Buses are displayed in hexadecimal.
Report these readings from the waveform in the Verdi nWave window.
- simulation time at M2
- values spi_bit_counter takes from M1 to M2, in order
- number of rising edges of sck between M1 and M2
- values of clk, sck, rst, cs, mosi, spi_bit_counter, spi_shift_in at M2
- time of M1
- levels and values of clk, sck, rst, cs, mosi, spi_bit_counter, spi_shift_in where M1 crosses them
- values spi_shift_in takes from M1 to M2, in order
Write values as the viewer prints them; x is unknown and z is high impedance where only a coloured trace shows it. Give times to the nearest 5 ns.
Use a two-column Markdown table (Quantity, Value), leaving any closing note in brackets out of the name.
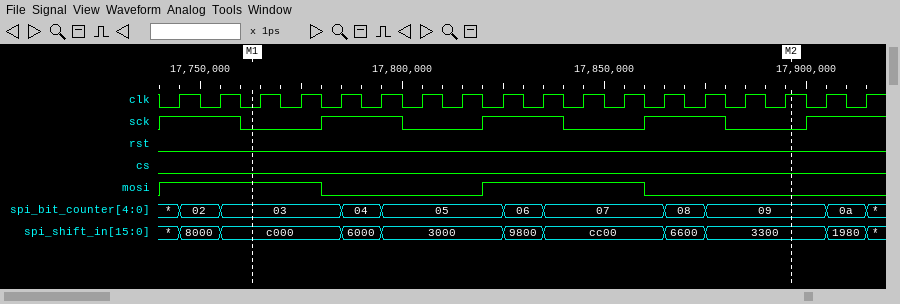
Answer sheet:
| Quantity | Value |
|---|---|
| simulation time at M2 | 17895 ns |
| values spi_bit_counter takes from M1 to M2, in order | 03, 04, 05, 06, 07, 08, 09 |
| number of rising edges of sck between M1 and M2 | 3 |
| values of clk, sck, rst, cs, mosi, spi_bit_counter, spi_shift_in at M2 | clk=1, sck=0, rst=0, cs=0, mosi=0, spi_bit_counter=09, spi_shift_in=3300 |
| time of M1 | 17765 ns |
| levels and values of clk, sck, rst, cs, mosi, spi_bit_counter, spi_shift_in where M1 crosses them | clk=0, sck=0, rst=0, cs=0, mosi=1, spi_bit_counter=03, spi_shift_in=c000 |
| values spi_shift_in takes from M1 to M2, in order | c000, 6000, 3000, 9800, cc00, 6600, 3300 |
